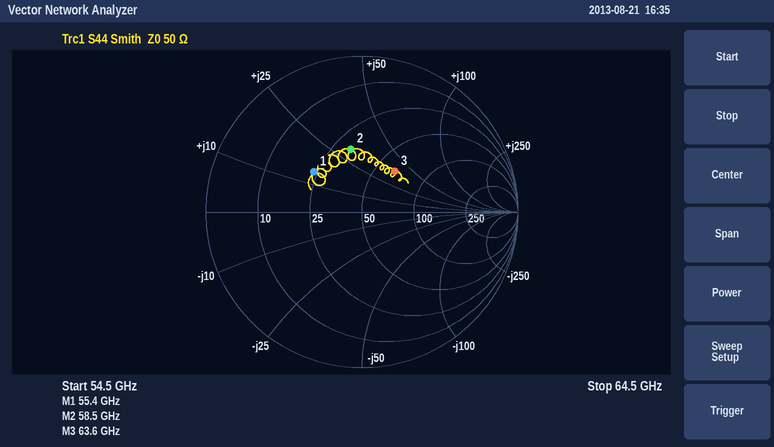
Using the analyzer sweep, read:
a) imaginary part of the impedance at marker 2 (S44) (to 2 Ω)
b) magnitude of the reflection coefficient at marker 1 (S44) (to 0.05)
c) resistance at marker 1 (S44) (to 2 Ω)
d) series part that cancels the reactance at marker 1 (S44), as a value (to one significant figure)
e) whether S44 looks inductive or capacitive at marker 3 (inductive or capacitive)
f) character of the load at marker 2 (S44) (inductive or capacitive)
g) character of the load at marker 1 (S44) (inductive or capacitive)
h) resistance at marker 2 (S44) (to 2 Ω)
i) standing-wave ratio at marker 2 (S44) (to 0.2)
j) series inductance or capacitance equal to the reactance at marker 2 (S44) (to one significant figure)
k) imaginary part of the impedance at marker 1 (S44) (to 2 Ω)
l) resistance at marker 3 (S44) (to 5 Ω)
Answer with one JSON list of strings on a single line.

["+30 Ω", "0.40", "24 Ω", "200 fF", "inductive", "inductive", "inductive", "32 Ω", "2.4", "80 pH", "+14 Ω", "65 Ω"]
